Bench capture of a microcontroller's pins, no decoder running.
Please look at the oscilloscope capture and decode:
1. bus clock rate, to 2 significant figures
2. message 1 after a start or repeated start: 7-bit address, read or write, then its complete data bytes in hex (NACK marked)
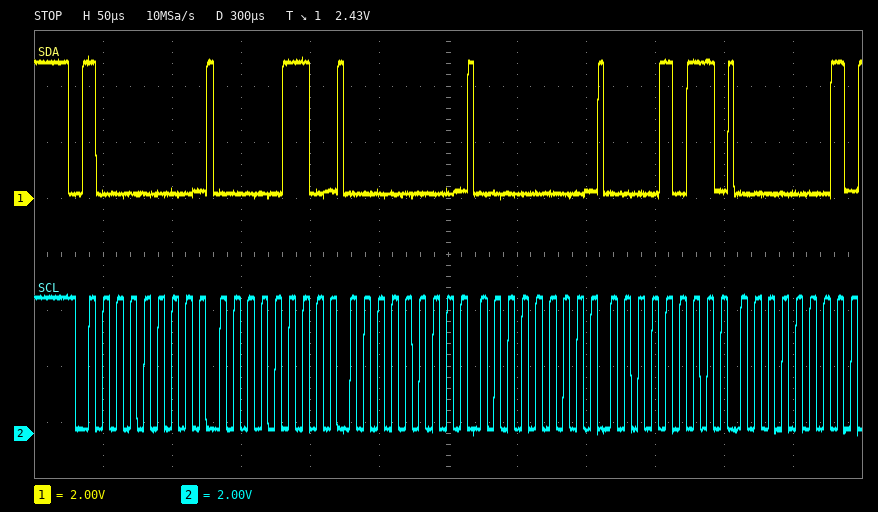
100 kHz
0x40 write: 06 00 00 0B 01
